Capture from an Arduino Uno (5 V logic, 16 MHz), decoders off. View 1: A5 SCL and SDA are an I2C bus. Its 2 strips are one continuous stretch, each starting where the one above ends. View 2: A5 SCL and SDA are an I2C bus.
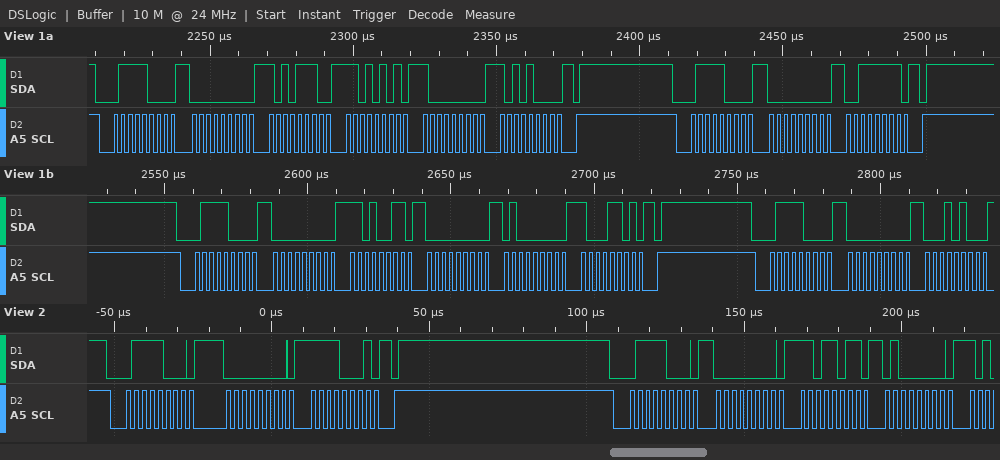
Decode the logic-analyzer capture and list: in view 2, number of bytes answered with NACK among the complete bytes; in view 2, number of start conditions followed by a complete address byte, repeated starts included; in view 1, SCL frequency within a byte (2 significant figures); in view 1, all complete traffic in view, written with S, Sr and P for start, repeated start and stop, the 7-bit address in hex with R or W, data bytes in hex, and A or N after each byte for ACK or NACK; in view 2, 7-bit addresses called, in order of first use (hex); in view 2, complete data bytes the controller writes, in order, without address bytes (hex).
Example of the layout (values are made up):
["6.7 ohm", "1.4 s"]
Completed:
["0", "2", "400 kHz", "S 3CW A 00 A AE A D5 A 80 A A8 A P S 3CW A 00 A 3F A P S 3CW A 00 A D3 A 00 A 40 A 8D A P S 3CW A 00 A 14 A", "0x3C", "00 F1 00 DB 40"]
